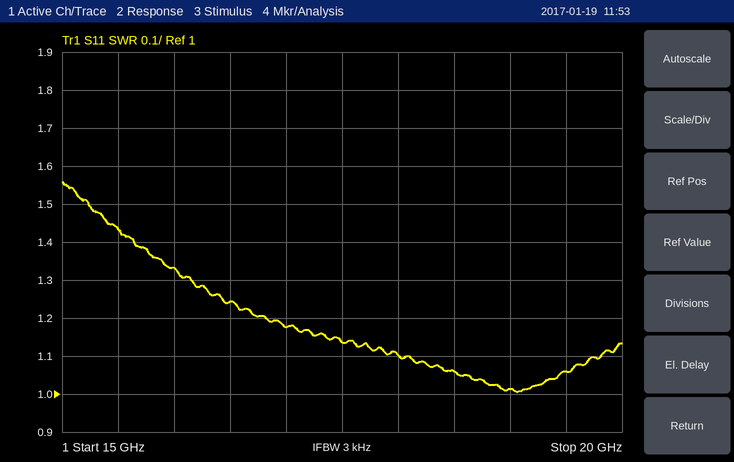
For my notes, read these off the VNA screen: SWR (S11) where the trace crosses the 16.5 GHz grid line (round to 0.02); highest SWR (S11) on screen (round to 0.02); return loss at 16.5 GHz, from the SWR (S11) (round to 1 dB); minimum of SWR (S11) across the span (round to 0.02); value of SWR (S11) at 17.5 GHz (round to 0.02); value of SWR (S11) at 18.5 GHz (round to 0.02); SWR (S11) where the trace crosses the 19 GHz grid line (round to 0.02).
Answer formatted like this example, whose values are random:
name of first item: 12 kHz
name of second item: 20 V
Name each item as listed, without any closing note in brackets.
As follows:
SWR (S11) where the trace crosses the 16.5 GHz grid line: 1.24
highest SWR (S11) on screen: 1.56
return loss at 16.5 GHz, from the SWR (S11): 19 dB
minimum of SWR (S11) across the span: 1.00
value of SWR (S11) at 17.5 GHz: 1.14
value of SWR (S11) at 18.5 GHz: 1.06
SWR (S11) where the trace crosses the 19 GHz grid line: 1.02
